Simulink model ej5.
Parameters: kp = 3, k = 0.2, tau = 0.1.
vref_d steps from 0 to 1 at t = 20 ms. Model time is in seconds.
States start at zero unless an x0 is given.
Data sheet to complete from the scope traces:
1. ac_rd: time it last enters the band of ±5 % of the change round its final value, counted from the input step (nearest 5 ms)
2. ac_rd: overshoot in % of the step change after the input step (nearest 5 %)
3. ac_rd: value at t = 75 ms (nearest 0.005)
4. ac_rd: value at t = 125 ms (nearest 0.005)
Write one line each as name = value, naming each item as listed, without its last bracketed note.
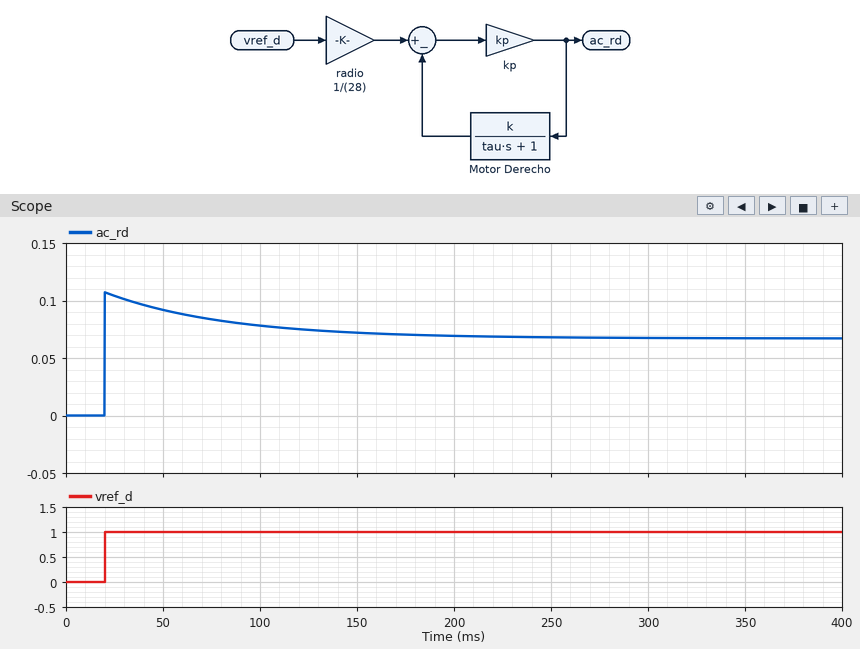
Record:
ac_rd: time it last enters the band of ±5 % of the change round its final value, counted from the input step = 155 ms
ac_rd: overshoot in % of the step change after the input step = 60 %
ac_rd: value at t = 75 ms = 0.085
ac_rd: value at t = 125 ms = 0.075
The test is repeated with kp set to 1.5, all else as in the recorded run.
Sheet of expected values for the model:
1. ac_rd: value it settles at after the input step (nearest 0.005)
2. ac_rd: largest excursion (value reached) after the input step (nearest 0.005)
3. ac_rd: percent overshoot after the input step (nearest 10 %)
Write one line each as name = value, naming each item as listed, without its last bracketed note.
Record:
ac_rd: value it settles at after the input step = 0.040
ac_rd: largest excursion (value reached) after the input step = 0.055
ac_rd: percent overshoot after the input step = 30 %
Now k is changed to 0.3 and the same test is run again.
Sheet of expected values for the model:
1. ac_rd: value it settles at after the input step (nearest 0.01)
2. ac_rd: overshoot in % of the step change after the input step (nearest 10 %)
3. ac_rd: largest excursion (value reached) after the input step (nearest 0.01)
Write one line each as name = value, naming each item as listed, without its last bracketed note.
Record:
ac_rd: value it settles at after the input step = 0.06
ac_rd: overshoot in % of the step change after the input step = 90 %
ac_rd: largest excursion (value reached) after the input step = 0.11
